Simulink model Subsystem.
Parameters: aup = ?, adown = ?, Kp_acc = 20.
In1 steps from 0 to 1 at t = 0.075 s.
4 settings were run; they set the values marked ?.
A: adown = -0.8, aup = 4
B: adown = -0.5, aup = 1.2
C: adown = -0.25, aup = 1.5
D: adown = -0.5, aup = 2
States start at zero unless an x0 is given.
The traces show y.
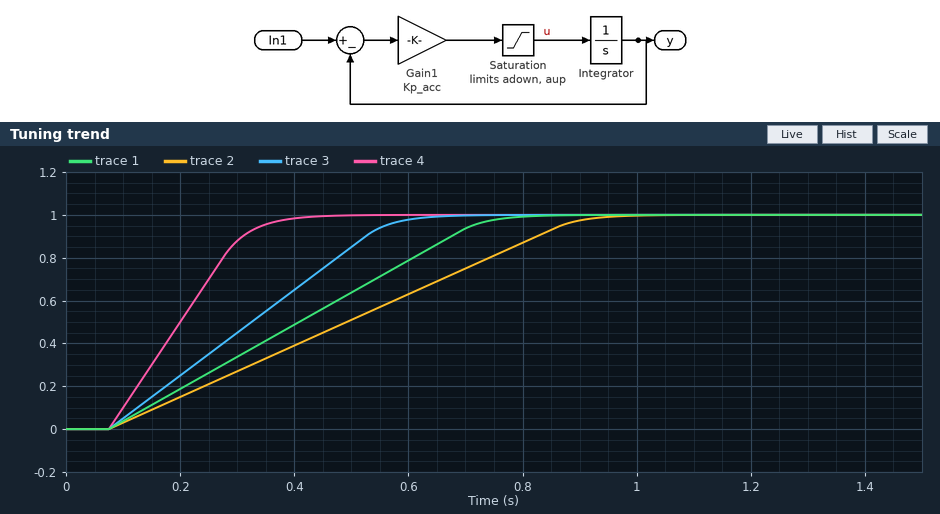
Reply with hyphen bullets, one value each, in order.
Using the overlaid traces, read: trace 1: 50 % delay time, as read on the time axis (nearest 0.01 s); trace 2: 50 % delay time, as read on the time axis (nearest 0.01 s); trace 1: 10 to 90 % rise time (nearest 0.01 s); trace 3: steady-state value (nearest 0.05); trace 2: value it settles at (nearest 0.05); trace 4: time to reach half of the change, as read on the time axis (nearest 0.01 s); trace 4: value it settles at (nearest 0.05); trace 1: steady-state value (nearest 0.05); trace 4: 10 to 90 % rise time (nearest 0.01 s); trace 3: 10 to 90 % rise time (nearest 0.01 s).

- 0.41 s
- 0.49 s
- 0.53 s
- 1.00
- 1.00
- 0.20 s
- 1.00
- 1.00
- 0.21 s
- 0.40 s
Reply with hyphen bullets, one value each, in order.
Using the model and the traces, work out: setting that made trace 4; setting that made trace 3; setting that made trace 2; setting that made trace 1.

- A
- D
- B
- C
